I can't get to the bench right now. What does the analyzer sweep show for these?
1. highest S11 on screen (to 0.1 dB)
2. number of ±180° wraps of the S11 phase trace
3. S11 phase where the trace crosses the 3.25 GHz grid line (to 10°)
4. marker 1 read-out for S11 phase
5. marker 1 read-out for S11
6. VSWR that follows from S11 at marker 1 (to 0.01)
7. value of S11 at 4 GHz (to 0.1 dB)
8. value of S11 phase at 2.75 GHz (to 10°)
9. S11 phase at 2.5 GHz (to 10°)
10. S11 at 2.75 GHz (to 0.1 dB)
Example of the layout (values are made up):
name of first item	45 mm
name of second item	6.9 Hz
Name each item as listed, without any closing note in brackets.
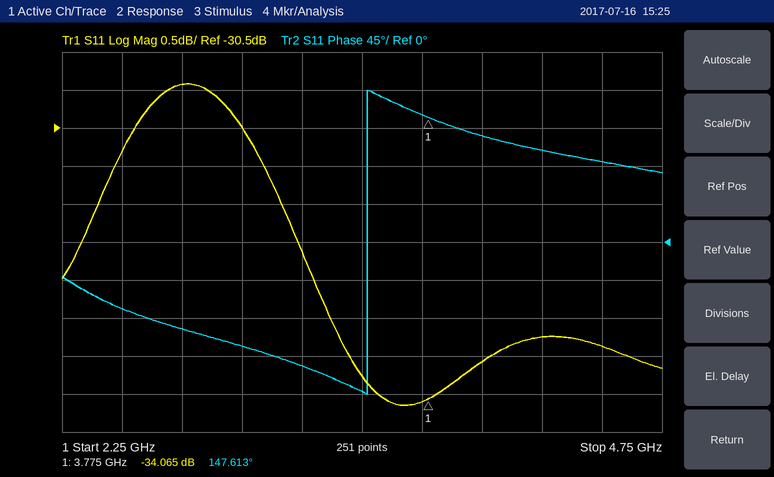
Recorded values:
highest S11 on screen	-29.9 dB
number of ±180° wraps of the S11 phase trace	1
S11 phase where the trace crosses the 3.25 GHz grid line	-150°
marker 1 read-out for S11 phase	147.613°
marker 1 read-out for S11	-34.065 dB
VSWR that follows from S11 at marker 1	1.04
value of S11 at 4 GHz	-33.6 dB
value of S11 phase at 2.75 GHz	-100°
S11 phase at 2.5 GHz	-80°
S11 at 2.75 GHz	-29.9 dB
